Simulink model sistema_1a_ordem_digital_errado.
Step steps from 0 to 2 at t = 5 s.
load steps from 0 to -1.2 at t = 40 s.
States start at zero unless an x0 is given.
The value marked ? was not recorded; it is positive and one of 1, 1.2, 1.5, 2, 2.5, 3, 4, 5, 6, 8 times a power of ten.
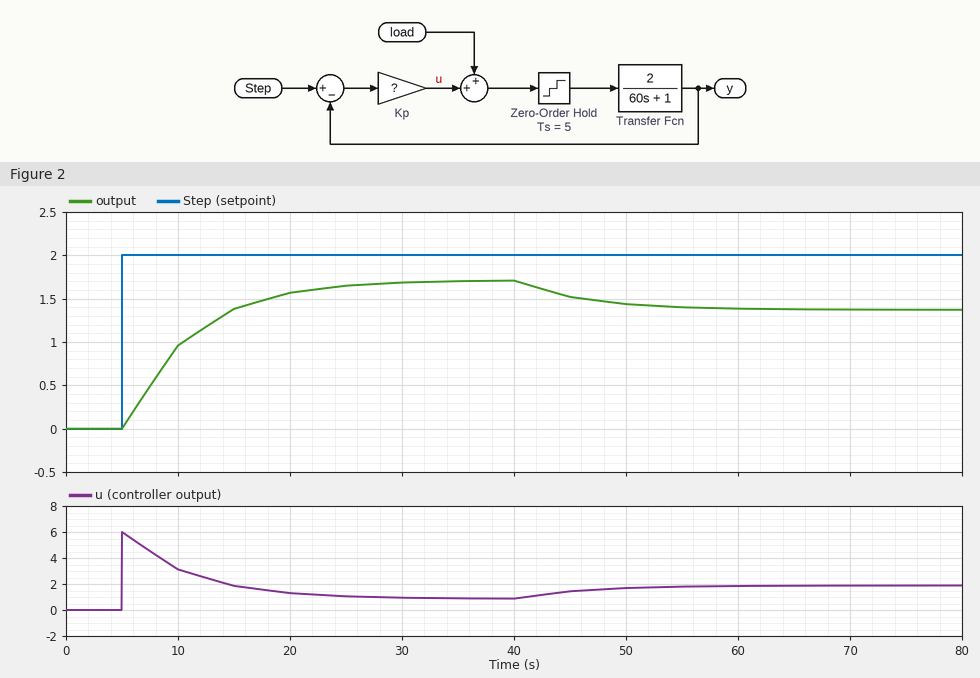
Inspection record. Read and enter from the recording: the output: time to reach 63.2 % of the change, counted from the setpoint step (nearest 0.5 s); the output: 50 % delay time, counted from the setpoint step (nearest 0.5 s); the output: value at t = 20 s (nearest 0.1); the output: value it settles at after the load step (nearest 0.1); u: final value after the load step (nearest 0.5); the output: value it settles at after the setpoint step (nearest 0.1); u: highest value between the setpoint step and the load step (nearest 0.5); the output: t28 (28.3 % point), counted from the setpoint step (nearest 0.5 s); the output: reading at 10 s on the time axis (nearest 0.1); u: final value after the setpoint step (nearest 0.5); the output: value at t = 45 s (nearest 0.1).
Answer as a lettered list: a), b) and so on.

a) 6.5 s
b) 4.5 s
c) 1.6
d) 1.4
e) 2.0
f) 1.7
g) 6.0
h) 2.5 s
i) 1.0
j) 1.0
k) 1.5
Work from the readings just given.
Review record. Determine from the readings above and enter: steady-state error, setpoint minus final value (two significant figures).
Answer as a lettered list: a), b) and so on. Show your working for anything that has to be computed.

a) 2 - 1.7 = 0.30
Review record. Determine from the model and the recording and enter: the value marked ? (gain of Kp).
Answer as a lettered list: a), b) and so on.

a) 3
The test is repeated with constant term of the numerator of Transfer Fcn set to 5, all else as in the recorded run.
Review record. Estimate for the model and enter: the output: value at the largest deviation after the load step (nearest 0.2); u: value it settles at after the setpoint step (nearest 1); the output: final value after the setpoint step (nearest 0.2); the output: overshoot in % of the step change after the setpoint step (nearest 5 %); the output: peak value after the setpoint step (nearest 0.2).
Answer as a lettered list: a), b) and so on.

a) 1.4
b) 0
c) 1.8
d) 30 %
e) 2.4
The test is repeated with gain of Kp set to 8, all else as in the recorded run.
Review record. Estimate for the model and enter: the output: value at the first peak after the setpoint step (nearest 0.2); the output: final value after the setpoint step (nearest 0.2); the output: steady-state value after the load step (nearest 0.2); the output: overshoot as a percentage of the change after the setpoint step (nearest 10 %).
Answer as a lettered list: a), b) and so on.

a) 2.6
b) 1.8
c) 1.8
d) 40 %
